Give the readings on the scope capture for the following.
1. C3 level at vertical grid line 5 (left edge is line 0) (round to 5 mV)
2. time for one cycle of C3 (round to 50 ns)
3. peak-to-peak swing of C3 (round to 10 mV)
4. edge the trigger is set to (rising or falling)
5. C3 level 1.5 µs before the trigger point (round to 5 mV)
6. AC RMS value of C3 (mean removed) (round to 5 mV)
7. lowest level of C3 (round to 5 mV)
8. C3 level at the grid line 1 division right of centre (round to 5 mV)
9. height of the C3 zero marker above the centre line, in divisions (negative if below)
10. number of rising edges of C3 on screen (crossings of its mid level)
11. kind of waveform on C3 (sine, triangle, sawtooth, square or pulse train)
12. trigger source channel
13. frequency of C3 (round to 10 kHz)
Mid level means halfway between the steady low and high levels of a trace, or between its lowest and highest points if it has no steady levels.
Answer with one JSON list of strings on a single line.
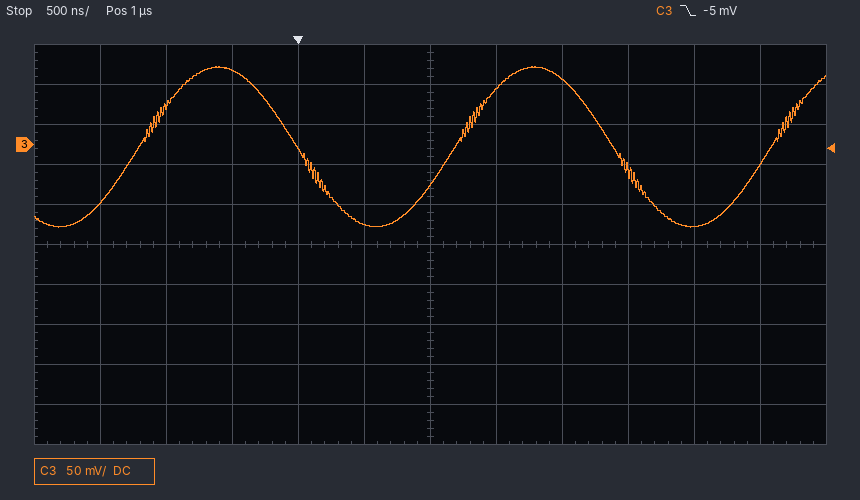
["-100 mV", "2.40 µs", "200 mV", "falling", "-75 mV", "70 mV", "-105 mV", "70 mV", "+2.5 div", "3", "sine", "C3", "420 kHz"]
